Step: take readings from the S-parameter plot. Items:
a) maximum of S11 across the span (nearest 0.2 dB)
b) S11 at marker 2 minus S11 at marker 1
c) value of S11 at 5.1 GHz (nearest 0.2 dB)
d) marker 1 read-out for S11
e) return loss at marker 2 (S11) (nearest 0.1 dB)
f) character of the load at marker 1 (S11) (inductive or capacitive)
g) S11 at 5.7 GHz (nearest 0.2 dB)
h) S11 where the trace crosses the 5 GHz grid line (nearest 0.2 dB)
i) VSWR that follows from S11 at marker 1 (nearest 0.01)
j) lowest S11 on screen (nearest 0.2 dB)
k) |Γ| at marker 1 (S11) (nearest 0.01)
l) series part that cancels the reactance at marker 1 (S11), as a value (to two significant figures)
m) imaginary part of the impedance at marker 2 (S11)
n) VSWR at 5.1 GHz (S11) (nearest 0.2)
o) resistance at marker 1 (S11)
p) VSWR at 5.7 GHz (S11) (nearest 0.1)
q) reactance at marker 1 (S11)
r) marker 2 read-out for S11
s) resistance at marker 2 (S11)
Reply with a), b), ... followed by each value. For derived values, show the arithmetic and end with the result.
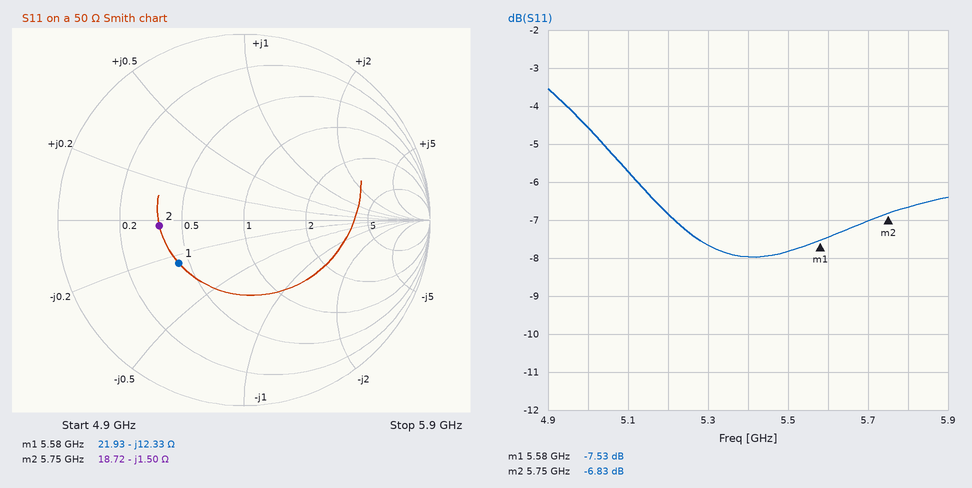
a) -3.6 dB
b) -6.83 − (-7.53) = 0.70 dB
c) -5.8 dB
d) -7.53 dB
e) 6.8 dB
f) capacitive
g) -7.0 dB
h) -4.6 dB
i) (1 + 0.4202)/(1 − 0.4202) ≈ 2.45
j) -8.0 dB
k) 0.42
l) L = 12.33 Ω/(2π × 5.58 GHz) ≈ 352 pH, so 350 pH to two significant figures
m) -1.50 Ω
n) |Γ| = 10^(-5.8/20) = 0.5129; VSWR = (1 + 0.5129)/(1 − 0.5129) ≈ 3.11, so 3.2 to the nearest 0.2
o) 21.93 Ω
p) |Γ| = 10^(-7/20) = 0.4467; VSWR = (1 + 0.4467)/(1 − 0.4467) ≈ 2.6
q) -12.33 Ω
r) -6.83 dB
s) 18.72 Ω
